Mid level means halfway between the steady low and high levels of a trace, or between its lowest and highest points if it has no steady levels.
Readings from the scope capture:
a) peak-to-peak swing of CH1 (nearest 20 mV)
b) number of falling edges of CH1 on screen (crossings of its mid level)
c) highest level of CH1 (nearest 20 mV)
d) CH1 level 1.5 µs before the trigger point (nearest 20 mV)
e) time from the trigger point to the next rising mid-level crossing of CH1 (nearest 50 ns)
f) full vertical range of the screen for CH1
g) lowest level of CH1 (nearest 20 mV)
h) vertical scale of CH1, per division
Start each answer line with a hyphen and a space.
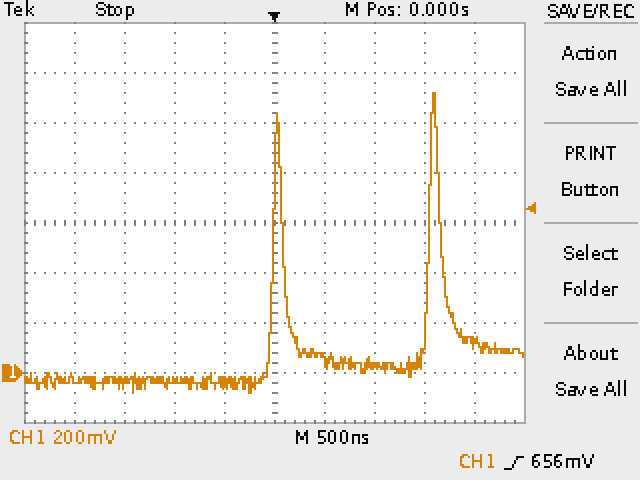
- 1.20 V
- 2
- 1.12 V
- -40 mV
- 1.55 µs
- 1.6 V
- -80 mV
- 200 mV
